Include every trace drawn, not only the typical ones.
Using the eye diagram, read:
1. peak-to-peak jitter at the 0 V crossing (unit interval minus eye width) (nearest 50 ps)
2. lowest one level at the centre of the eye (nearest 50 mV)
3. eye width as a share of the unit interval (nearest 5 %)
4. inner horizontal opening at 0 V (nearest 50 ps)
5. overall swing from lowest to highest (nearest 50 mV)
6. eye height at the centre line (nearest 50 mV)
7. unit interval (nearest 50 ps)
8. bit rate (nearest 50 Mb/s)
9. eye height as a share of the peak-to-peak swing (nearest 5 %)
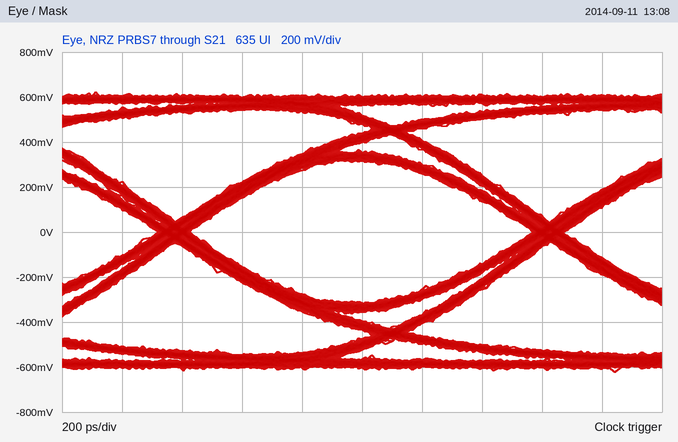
100 ps
300 mV
90 %
1.15 ns
1.25 V
650 mV
1.25 ns
800 Mb/s
50 %
